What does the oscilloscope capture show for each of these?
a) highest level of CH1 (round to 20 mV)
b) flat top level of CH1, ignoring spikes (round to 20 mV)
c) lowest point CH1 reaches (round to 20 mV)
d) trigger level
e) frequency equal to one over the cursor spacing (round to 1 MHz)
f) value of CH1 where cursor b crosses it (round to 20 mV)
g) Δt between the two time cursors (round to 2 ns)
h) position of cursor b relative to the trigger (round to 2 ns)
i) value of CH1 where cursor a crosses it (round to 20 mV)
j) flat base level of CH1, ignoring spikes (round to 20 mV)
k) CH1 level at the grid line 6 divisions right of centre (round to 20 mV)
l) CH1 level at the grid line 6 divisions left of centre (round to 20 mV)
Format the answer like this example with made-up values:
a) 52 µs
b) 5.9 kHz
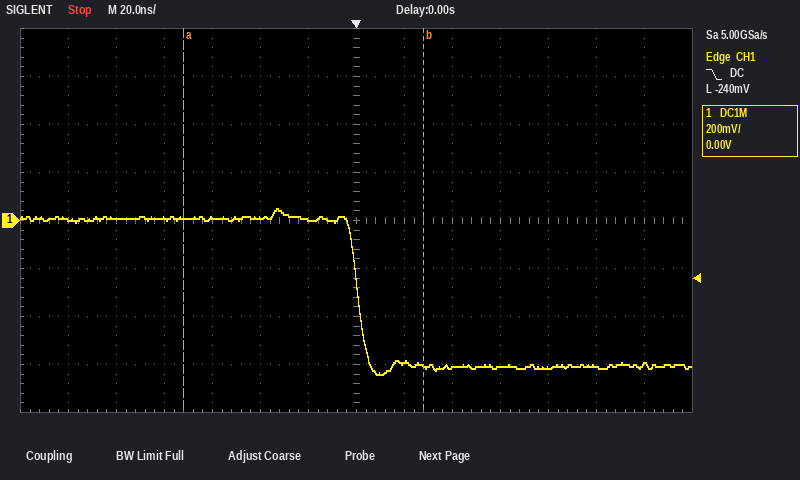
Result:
a) 40 mV
b) 0 mV
c) -640 mV
d) -240 mV
e) 10 MHz
f) -600 mV
g) 100 ns
h) +28 ns
i) 20 mV
j) -600 mV
k) -600 mV
l) 0 mV
